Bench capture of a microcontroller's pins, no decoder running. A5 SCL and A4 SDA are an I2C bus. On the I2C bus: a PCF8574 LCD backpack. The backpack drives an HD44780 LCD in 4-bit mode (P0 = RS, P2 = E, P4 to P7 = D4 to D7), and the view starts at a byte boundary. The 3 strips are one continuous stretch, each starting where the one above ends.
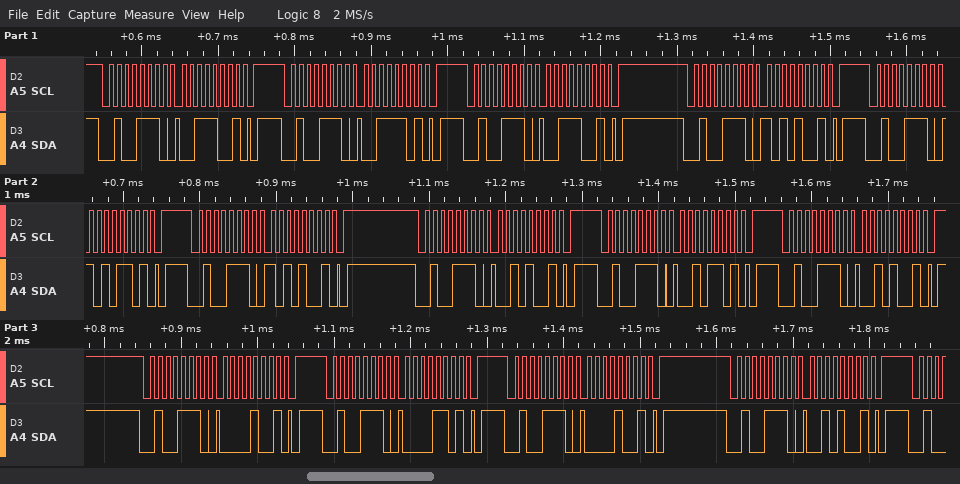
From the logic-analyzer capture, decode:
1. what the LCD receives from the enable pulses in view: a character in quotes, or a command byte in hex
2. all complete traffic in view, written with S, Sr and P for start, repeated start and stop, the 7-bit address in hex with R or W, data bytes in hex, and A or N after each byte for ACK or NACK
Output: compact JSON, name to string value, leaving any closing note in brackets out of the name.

{"what the LCD receives from the enable pulses in view: a character in quotes, or a command byte in hex": "':' ' '", "all complete traffic in view, written with S, Sr and P for start, repeated start and stop, the 7-bit address in hex with R or W, data bytes in hex, and A or N after each byte for ACK or NACK": "S 27W A 39 A P S 27W A 3D A P S 27W A 39 A P S 27W A A9 A P S 27W A AD A P S 27W A A9 A P S 27W A 29 A P S 27W A 2D A P S 27W A 29 A P S 27W A 09 A P S 27W A 0D A P S 27W A 09 A P S 27W A 29 A P"}
